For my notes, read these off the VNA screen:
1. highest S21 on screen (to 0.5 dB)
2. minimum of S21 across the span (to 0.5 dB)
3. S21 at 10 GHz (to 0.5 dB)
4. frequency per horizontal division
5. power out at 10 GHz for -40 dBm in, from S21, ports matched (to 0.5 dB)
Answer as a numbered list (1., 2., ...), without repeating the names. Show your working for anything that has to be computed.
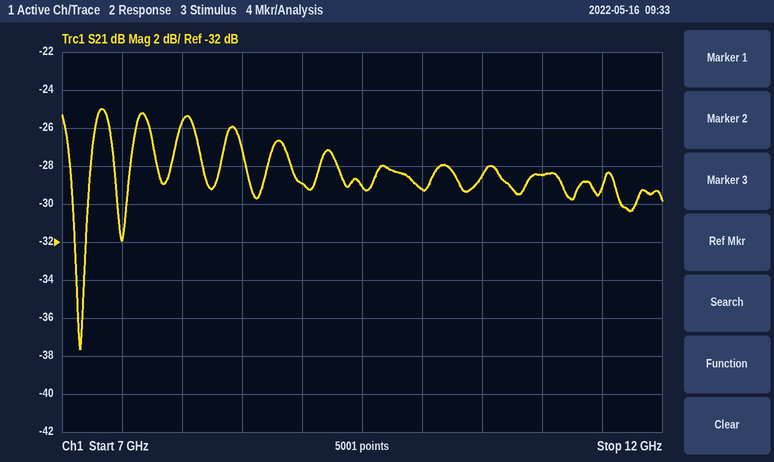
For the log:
1. -25.0 dB
2. -37.5 dB
3. -29.0 dB
4. 500 MHz
5. -40 dBm + (-29.0 dB) = -69.0 dBm
